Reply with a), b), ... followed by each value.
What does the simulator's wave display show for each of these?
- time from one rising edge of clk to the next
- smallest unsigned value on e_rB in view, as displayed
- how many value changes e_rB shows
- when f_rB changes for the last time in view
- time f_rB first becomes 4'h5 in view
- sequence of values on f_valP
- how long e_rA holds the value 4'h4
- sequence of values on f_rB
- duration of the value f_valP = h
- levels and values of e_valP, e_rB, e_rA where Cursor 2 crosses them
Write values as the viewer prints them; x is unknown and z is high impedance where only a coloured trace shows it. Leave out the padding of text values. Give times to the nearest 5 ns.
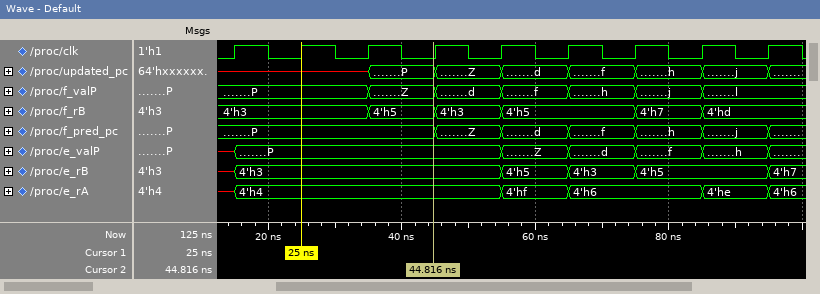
a) 10 ns
b) 4'h3
c) 5
d) 85 ns
e) 35 ns
f) P, Z, d, f, h, j, l
g) 40 ns
h) 4'h3, 4'h5, 4'h3, 4'h5, 4'h7, 4'hd
i) 10 ns
j) e_valP=P, e_rB=4'h3, e_rA=4'h4
